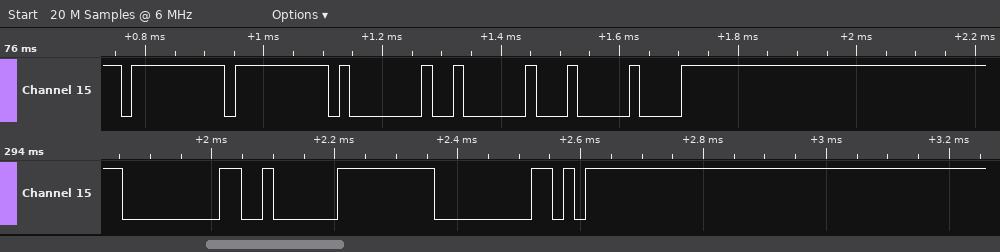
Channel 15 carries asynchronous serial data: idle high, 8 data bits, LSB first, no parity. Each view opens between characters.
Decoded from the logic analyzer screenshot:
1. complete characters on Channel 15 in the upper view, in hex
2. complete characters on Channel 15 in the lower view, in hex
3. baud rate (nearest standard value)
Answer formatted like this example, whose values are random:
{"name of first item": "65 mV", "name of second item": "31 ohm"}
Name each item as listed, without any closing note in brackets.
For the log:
{"complete characters on Channel 15 in the upper view, in hex": "FF, FF, 01, 02, 04, F8", "complete characters on Channel 15 in the lower view, in hex": "00, 02, 00, FD", "baud rate": "57600 baud"}
